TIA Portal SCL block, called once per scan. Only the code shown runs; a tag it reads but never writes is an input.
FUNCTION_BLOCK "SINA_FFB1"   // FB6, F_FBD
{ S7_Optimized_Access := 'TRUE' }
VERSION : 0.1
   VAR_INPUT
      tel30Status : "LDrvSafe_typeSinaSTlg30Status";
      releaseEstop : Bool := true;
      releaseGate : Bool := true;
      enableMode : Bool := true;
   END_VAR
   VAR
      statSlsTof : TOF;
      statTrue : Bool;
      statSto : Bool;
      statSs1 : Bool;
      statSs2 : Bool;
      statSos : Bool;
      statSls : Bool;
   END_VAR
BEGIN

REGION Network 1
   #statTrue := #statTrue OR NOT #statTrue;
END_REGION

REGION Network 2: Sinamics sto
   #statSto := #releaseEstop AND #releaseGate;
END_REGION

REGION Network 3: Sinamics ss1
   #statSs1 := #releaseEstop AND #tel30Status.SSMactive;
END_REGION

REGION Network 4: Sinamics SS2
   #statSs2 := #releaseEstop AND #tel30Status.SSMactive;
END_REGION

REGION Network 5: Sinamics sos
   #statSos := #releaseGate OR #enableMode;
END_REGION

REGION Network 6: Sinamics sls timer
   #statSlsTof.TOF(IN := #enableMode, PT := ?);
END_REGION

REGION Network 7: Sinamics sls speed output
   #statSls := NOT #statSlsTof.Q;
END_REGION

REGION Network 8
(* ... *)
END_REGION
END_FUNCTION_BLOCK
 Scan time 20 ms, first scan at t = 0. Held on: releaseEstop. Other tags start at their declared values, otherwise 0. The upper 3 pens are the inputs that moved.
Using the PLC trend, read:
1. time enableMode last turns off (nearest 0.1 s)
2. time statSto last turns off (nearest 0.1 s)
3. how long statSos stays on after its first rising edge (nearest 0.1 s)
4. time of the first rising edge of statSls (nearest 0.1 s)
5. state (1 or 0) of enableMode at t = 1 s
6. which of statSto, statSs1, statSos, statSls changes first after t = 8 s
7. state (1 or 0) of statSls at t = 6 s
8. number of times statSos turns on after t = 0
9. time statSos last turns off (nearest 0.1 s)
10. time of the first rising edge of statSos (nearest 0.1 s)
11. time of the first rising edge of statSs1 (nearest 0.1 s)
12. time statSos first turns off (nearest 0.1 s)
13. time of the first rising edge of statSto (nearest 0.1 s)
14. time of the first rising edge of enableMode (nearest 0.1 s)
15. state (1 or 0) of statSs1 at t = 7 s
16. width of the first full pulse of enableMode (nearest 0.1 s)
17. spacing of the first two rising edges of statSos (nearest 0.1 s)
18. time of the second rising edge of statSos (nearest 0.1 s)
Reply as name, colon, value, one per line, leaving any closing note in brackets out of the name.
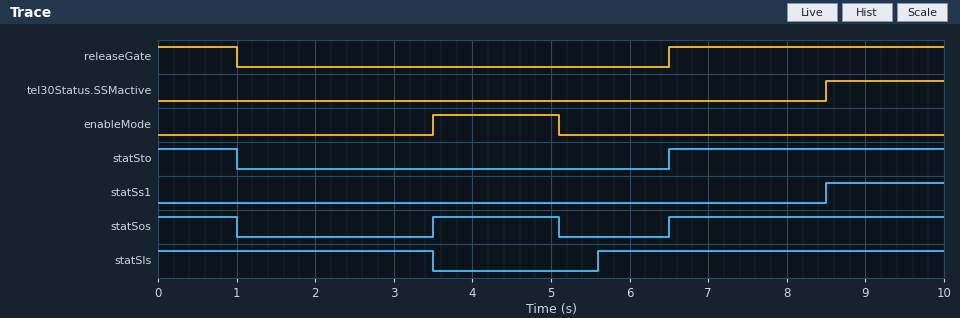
time enableMode last turns off: 5.1 s
time statSto last turns off: 1.0 s
how long statSos stays on after its first rising edge: 1.6 s
time of the first rising edge of statSls: 5.6 s
state (1 or 0) of enableMode at t = 1 s: 0
which of statSto, statSs1, statSos, statSls changes first after t = 8 s: statSs1
state (1 or 0) of statSls at t = 6 s: 1
number of times statSos turns on after t = 0: 2
time statSos last turns off: 5.1 s
time of the first rising edge of statSos: 3.5 s
time of the first rising edge of statSs1: 8.5 s
time statSos first turns off: 1.0 s
time of the first rising edge of statSto: 6.5 s
time of the first rising edge of enableMode: 3.5 s
state (1 or 0) of statSs1 at t = 7 s: 0
width of the first full pulse of enableMode: 1.6 s
spacing of the first two rising edges of statSos: 3.0 s
time of the second rising edge of statSos: 6.5 s
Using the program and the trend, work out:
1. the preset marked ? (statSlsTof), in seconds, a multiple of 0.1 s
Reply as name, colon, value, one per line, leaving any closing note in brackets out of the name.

the preset marked ? (statSlsTof), in seconds, a multiple of 0.1 s: 0.5 s
